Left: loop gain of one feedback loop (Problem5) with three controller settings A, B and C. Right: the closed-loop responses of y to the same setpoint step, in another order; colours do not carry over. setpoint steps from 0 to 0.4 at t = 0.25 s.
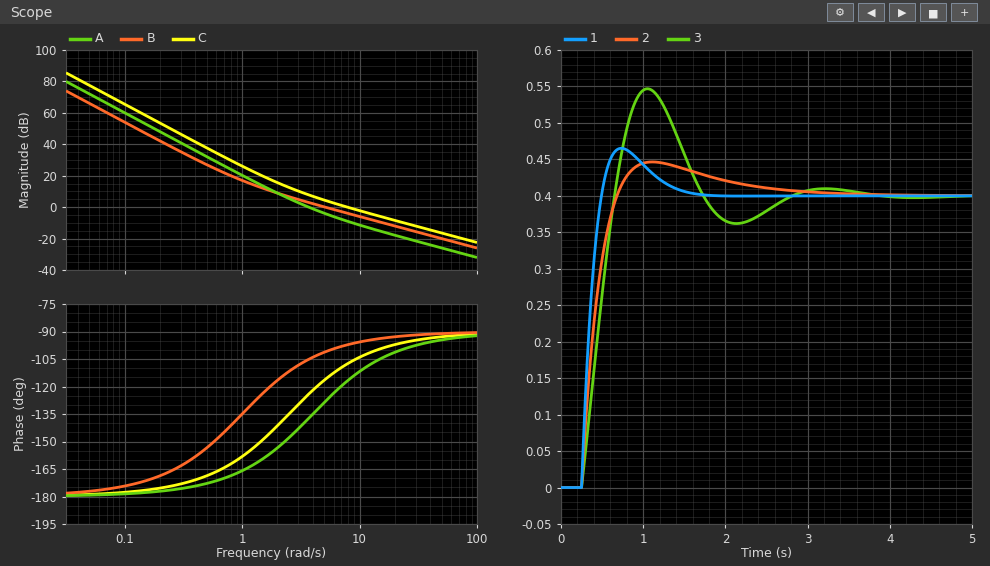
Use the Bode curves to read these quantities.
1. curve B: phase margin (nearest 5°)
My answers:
80°
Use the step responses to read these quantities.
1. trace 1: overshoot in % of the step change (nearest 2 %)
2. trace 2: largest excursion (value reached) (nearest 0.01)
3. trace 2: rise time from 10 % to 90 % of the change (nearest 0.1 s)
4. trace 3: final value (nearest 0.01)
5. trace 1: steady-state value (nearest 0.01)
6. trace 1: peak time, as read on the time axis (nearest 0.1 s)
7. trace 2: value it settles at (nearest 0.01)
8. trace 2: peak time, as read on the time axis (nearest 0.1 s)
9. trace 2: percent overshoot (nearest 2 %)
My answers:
16 %
0.45
0.3 s
0.40
0.40
0.7 s
0.40
1.1 s
12 %
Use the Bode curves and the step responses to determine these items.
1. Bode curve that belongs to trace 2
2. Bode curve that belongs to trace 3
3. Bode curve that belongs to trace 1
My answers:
B
A
C
